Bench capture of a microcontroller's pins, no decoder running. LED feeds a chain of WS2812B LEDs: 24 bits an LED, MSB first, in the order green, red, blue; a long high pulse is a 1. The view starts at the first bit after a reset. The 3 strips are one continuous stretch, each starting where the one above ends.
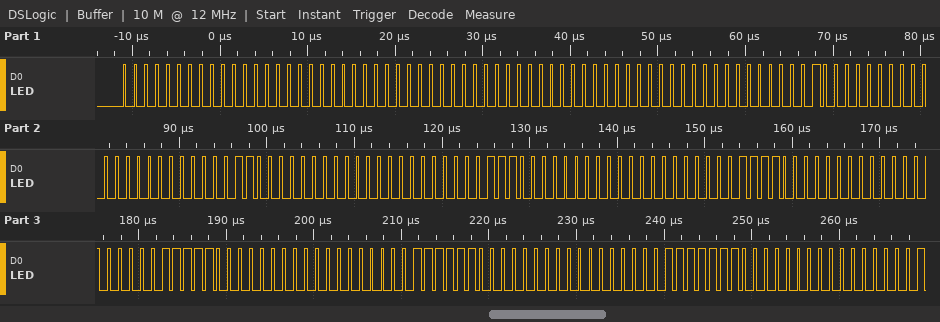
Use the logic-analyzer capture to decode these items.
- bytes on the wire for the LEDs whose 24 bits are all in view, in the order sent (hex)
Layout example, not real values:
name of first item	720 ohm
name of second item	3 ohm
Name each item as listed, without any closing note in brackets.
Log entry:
bytes on the wire for the LEDs whose 24 bits are all in view, in the order sent	00 00 00 00 00 00 00 01 00 00 03 00 00 07 00 00 0F 00 00 1F 00 00 3F 00 00 7F 00
